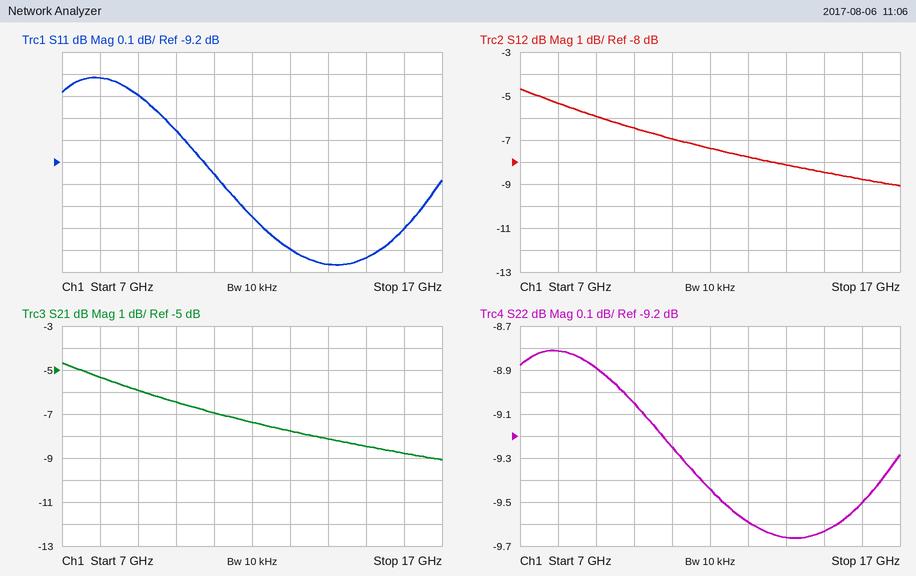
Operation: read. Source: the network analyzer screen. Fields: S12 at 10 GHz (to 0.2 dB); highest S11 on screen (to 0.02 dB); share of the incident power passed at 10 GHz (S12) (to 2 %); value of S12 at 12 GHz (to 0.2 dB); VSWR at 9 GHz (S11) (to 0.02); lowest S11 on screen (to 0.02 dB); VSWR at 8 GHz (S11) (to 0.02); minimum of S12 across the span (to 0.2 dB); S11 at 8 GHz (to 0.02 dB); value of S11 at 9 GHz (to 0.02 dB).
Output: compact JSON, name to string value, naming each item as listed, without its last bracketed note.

{"S12 at 10 GHz": "-6.4 dB", "highest S11 on screen": "-8.82 dB", "share of the incident power passed at 10 GHz (S12)": "22 %", "value of S12 at 12 GHz": "-7.4 dB", "VSWR at 9 GHz (S11)": "2.12", "lowest S11 on screen": "-9.66 dB", "VSWR at 8 GHz (S11)": "2.14", "minimum of S12 across the span": "-9.0 dB", "S11 at 8 GHz": "-8.82 dB", "value of S11 at 9 GHz": "-8.90 dB"}
